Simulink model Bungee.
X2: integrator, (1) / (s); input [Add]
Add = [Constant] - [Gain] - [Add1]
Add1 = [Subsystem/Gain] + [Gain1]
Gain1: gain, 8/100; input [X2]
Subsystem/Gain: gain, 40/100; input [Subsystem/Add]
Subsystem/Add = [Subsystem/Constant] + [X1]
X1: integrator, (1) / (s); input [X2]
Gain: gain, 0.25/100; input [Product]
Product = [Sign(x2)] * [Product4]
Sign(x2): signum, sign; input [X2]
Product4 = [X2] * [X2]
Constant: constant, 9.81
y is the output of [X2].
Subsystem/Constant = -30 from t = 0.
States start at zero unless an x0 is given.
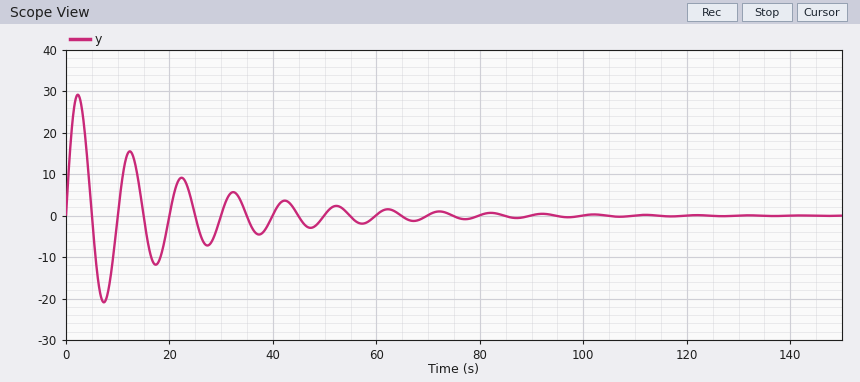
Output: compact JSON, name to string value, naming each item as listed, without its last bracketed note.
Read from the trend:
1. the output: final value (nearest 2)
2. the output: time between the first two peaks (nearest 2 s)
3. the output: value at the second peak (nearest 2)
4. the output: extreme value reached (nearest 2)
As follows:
{"the output: final value": "0", "the output: time between the first two peaks": "10 s", "the output: value at the second peak": "16", "the output: extreme value reached": "30"}
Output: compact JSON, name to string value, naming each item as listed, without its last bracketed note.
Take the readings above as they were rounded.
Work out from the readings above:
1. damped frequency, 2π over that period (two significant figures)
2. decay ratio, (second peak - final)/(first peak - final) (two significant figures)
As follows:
{"damped frequency, 2π over that period": "0.63 rad/s", "decay ratio, (second peak - final)/(first peak - final)": "0.53"}
